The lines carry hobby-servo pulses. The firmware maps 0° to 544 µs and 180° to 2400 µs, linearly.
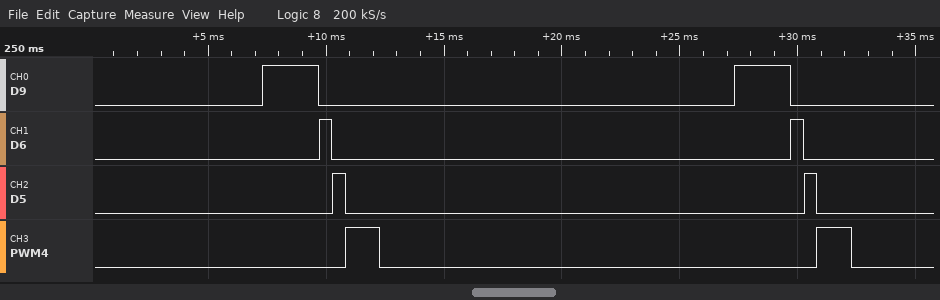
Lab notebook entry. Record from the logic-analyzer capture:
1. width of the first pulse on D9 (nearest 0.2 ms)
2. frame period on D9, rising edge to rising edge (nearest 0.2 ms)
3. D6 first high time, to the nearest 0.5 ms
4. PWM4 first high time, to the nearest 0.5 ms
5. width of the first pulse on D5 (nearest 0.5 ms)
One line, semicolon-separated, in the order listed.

2.4 ms; 20.0 ms; 0.5 ms; 1.5 ms; 0.5 ms
